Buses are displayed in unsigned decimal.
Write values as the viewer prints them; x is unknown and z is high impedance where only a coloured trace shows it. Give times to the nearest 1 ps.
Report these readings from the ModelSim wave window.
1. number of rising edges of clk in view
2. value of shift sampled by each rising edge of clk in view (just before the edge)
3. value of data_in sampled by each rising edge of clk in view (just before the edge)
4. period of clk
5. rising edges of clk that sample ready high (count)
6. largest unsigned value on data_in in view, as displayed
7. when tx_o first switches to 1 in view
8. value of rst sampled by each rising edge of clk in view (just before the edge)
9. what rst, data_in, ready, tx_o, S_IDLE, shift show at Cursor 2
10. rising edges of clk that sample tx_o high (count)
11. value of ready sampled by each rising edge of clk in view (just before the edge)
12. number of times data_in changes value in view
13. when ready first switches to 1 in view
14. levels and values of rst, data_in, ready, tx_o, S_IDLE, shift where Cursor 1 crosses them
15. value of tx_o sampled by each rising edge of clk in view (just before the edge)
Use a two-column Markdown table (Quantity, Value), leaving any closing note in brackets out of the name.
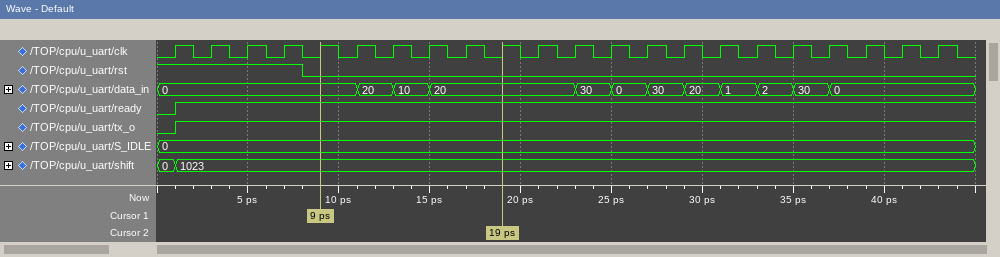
| Quantity | Value |
|---|---|
| number of rising edges of clk in view | 22 |
| value of shift sampled by each rising edge of clk in view | 0, 1023, 1023, 1023, 1023, 1023, 1023, 1023, 1023, 1023, 1023, 1023, 1023, 1023, 1023, 1023, 1023, 1023, 1023, 1023, 1023, 1023 |
| value of data_in sampled by each rising edge of clk in view | 0, 0, 0, 0, 0, 0, 20, 10, 20, 20, 20, 20, 30, 0, 30, 20, 1, 2, 30, 0, 0, 0 |
| period of clk | 2 ps |
| rising edges of clk that sample ready high | 21 |
| largest unsigned value on data_in in view, as displayed | 30 |
| when tx_o first switches to 1 in view | 1 ps |
| value of rst sampled by each rising edge of clk in view | 1 1 1 1 0 0 0 0 0 0 0 0 0 0 0 0 0 0 0 0 0 0 |
| what rst, data_in, ready, tx_o, S_IDLE, shift show at Cursor 2 | rst=0, data_in=20, ready=1, tx_o=1, S_IDLE=0, shift=1023 |
| rising edges of clk that sample tx_o high | 21 |
| value of ready sampled by each rising edge of clk in view | 0 1 1 1 1 1 1 1 1 1 1 1 1 1 1 1 1 1 1 1 1 1 |
| number of times data_in changes value in view | 11 |
| when ready first switches to 1 in view | 1 ps |
| levels and values of rst, data_in, ready, tx_o, S_IDLE, shift where Cursor 1 crosses them | rst=0, data_in=0, ready=1, tx_o=1, S_IDLE=0, shift=1023 |
| value of tx_o sampled by each rising edge of clk in view | 0 1 1 1 1 1 1 1 1 1 1 1 1 1 1 1 1 1 1 1 1 1 |
